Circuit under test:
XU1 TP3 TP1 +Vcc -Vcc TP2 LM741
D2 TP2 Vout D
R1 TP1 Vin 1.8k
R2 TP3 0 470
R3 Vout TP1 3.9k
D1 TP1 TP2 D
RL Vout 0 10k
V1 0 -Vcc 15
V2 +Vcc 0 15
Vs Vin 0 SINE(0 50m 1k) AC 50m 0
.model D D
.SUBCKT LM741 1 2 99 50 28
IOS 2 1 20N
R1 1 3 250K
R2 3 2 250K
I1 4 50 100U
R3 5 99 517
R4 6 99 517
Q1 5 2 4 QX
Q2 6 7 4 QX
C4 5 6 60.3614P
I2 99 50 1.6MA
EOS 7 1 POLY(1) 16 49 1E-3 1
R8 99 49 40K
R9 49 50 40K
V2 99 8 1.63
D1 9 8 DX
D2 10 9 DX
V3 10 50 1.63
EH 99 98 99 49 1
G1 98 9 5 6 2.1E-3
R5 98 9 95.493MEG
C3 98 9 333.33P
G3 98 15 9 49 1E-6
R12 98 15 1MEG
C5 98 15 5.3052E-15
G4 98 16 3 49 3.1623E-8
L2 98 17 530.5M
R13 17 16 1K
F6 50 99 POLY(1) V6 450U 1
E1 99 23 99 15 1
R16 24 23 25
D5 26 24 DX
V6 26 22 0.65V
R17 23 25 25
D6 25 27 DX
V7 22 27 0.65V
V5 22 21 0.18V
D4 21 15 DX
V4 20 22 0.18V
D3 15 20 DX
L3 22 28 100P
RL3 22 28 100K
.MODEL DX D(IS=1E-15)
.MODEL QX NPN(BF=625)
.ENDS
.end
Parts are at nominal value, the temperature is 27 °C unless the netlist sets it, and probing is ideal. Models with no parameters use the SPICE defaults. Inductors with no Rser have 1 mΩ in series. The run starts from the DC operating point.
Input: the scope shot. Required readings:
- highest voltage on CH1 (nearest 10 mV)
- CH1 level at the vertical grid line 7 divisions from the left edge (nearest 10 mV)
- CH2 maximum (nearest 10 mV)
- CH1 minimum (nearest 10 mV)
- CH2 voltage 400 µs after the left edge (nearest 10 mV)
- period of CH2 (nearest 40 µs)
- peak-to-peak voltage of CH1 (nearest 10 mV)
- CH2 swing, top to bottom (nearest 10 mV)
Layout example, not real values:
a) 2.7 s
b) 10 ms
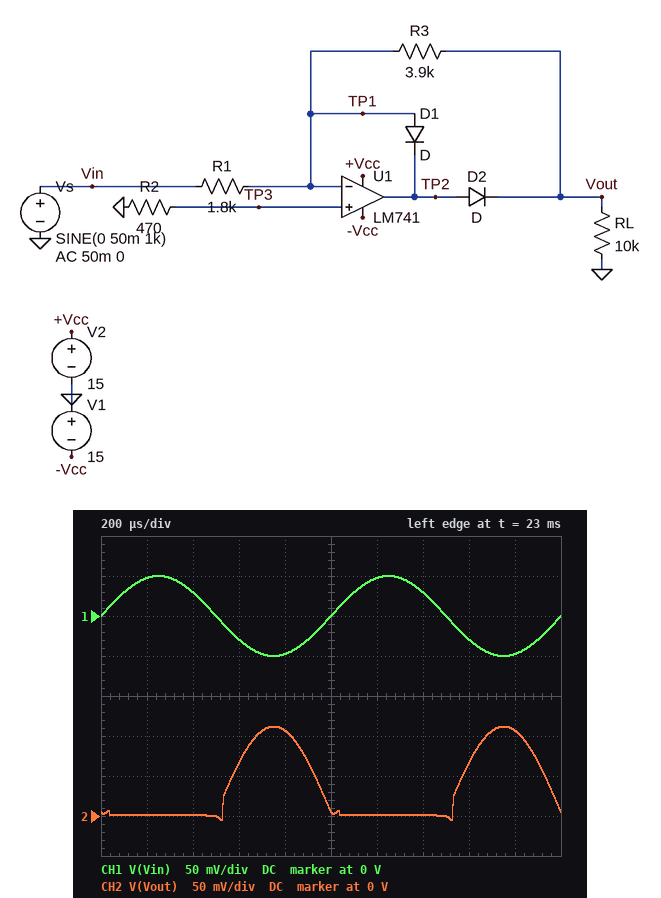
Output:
a) 50 mV
b) 30 mV
c) 110 mV
d) -50 mV
e) 0 V
f) 1.00 ms
g) 100 mV
h) 120 mV
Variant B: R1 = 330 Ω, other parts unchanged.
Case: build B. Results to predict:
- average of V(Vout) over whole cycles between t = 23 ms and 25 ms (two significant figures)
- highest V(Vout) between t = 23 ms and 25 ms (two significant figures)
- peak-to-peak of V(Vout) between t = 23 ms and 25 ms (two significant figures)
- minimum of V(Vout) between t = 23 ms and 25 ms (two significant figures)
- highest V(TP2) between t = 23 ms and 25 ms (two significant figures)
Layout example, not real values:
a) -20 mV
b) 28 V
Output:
a) 190 mV
b) 600 mV
c) 610 mV
d) -5.8 mV
e) 1.2 V
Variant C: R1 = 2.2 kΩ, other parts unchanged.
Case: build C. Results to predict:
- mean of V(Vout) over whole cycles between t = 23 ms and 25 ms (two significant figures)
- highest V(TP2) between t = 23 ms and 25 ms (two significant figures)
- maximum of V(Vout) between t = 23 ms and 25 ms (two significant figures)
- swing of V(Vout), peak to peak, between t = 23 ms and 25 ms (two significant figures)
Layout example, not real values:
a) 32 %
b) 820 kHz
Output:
a) 30 mV
b) 660 mV
c) 92 mV
d) 97 mV
